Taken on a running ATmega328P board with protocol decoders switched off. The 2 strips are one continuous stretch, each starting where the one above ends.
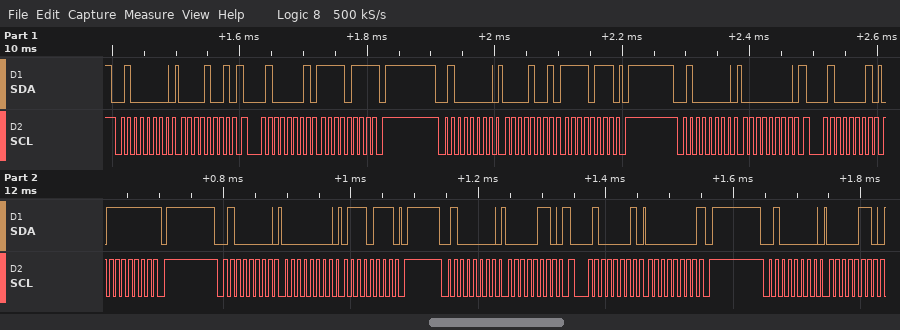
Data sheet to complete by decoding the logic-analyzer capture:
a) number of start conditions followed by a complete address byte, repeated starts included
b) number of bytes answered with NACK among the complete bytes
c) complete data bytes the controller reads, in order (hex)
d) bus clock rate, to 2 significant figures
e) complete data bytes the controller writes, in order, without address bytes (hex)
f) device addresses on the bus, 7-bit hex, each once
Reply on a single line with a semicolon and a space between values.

9; 3; F7 7F 00; 100 kHz; 09 09 F7 00 00 77 06 06; 0x20
